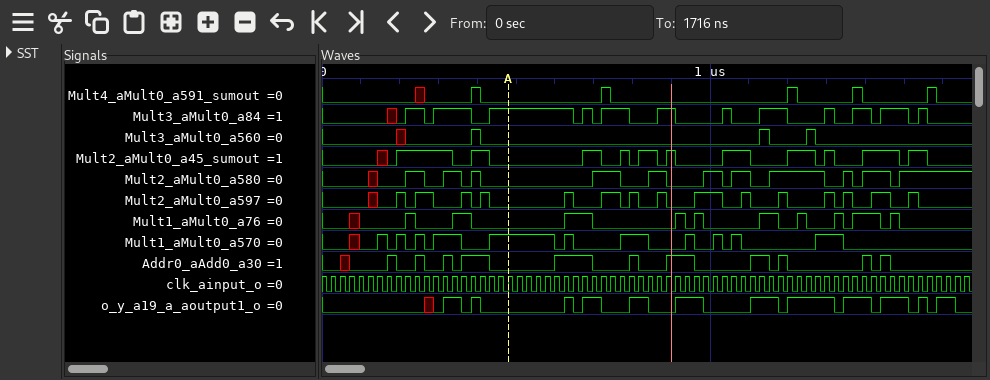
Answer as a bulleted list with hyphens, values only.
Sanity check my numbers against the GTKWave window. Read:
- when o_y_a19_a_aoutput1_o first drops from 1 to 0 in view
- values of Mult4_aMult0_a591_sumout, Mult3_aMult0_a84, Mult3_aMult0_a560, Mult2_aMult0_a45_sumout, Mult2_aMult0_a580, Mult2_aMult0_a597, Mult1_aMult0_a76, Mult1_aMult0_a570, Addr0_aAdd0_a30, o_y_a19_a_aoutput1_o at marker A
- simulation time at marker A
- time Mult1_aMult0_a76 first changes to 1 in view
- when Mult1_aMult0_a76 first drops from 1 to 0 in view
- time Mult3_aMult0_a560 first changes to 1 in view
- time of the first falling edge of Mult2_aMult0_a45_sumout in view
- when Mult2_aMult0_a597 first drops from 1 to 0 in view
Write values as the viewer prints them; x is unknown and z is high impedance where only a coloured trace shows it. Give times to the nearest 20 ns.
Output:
- 360 ns
- Mult4_aMult0_a591_sumout=0, Mult3_aMult0_a84=1, Mult3_aMult0_a560=0, Mult2_aMult0_a45_sumout=0, Mult2_aMult0_a580=0, Mult2_aMult0_a597=0, Mult1_aMult0_a76=0, Mult1_aMult0_a570=1, Addr0_aAdd0_a30=0, o_y_a19_a_aoutput1_o=0
- 480 ns
- 220 ns
- 240 ns
- 380 ns
- 340 ns
- 220 ns
